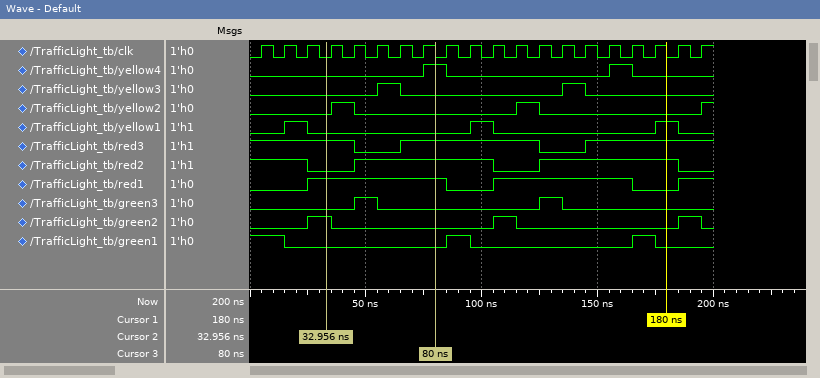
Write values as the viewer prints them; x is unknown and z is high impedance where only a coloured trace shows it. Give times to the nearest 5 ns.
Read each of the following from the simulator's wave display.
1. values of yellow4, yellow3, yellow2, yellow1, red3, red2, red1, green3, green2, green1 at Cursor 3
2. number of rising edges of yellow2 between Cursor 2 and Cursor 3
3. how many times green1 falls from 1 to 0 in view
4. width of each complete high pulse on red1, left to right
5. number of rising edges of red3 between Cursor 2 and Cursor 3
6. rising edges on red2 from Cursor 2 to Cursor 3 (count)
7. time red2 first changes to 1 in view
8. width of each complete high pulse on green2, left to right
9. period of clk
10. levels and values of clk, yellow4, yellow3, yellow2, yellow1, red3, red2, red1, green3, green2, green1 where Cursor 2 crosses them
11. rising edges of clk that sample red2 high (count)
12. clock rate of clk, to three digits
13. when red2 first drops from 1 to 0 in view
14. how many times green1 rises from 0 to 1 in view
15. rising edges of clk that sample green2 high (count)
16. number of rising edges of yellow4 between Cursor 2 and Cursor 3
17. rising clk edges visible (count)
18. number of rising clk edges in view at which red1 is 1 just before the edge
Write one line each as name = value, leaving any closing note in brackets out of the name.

values of yellow4, yellow3, yellow2, yellow1, red3, red2, red1, green3, green2, green1 at Cursor 3 = yellow4=1, yellow3=0, yellow2=0, yellow1=0, red3=1, red2=1, red1=1, green3=0, green2=0, green1=0
number of rising edges of yellow2 between Cursor 2 and Cursor 3 = 1
how many times green1 falls from 1 to 0 in view = 3
width of each complete high pulse on red1, left to right = 60 ns, 60 ns
number of rising edges of red3 between Cursor 2 and Cursor 3 = 1
rising edges on red2 from Cursor 2 to Cursor 3 = 1
time red2 first changes to 1 in view = 45 ns
width of each complete high pulse on green2, left to right = 10 ns, 10 ns, 10 ns
period of clk = 10 ns
levels and values of clk, yellow4, yellow3, yellow2, yellow1, red3, red2, red1, green3, green2, green1 where Cursor 2 crosses them = clk=0, yellow4=0, yellow3=0, yellow2=0, yellow1=0, red3=1, red2=0, red1=1, green3=0, green2=1, green1=0
rising edges of clk that sample red2 high = 15
clock rate of clk, to three digits = 100 MHz
when red2 first drops from 1 to 0 in view = 25 ns
how many times green1 rises from 0 to 1 in view = 2
rising edges of clk that sample green2 high = 3
number of rising edges of yellow4 between Cursor 2 and Cursor 3 = 1
rising clk edges visible = 20
number of rising clk edges in view at which red1 is 1 just before the edge = 13
